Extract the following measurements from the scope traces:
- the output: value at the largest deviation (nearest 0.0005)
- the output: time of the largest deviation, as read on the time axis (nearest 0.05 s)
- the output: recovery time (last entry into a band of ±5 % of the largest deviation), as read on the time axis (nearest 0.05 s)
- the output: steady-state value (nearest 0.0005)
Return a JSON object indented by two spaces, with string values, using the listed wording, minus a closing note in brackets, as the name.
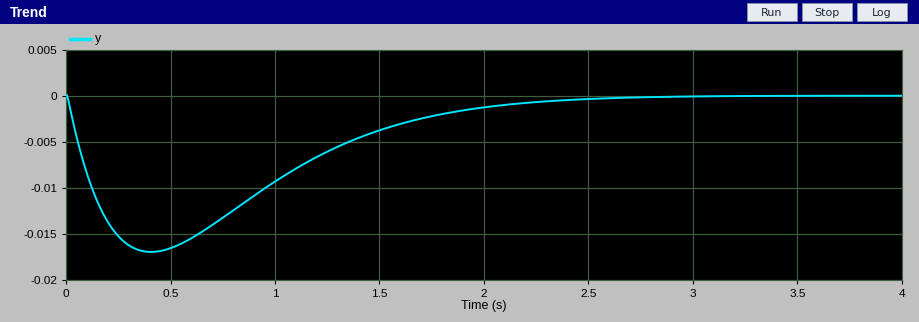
{
  "the output: value at the largest deviation": "-0.0170",
  "the output: time of the largest deviation, as read on the time axis": "0.40 s",
  "the output: recovery time (last entry into a band of ±5 % of the largest deviation), as read on the time axis": "2.15 s",
  "the output: steady-state value": "0.0000"
}
